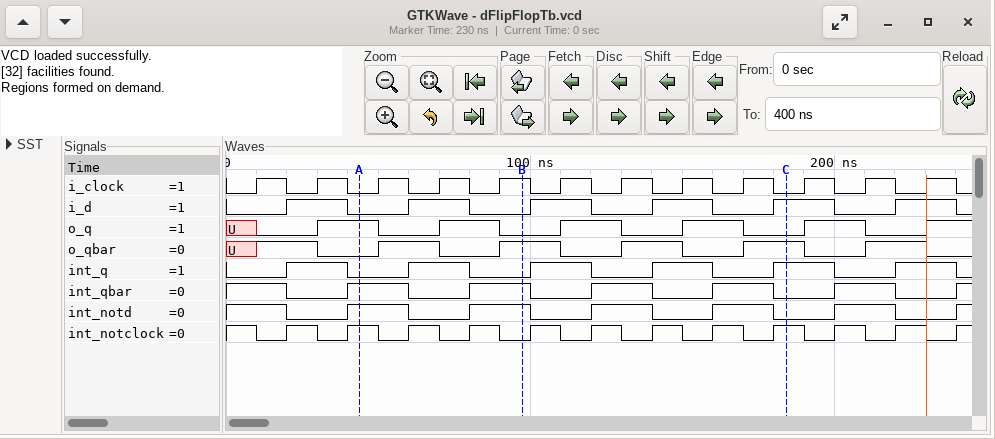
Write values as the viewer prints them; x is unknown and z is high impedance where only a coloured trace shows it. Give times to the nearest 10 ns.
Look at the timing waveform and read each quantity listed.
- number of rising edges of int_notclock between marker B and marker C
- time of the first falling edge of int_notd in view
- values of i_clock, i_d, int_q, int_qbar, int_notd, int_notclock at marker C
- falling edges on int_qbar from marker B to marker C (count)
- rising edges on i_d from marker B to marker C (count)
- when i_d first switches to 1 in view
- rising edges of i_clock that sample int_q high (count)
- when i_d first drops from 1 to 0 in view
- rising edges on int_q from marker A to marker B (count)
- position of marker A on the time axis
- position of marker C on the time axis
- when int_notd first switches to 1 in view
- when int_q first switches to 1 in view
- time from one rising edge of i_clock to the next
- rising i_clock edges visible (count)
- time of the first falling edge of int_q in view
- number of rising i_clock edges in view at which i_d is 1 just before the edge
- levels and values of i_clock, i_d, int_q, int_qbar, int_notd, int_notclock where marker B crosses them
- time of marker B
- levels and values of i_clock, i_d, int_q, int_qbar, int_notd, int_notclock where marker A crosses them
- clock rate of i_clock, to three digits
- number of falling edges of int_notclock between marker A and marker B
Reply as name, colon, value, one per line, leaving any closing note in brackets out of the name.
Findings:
number of rising edges of int_notclock between marker B and marker C: 5
time of the first falling edge of int_notd in view: 20 ns
values of i_clock, i_d, int_q, int_qbar, int_notd, int_notclock at marker C: i_clock=0, i_d=1, int_q=1, int_qbar=0, int_notd=0, int_notclock=1
falling edges on int_qbar from marker B to marker C: 3
rising edges on i_d from marker B to marker C: 3
when i_d first switches to 1 in view: 20 ns
rising edges of i_clock that sample int_q high: 6
when i_d first drops from 1 to 0 in view: 40 ns
rising edges on int_q from marker A to marker B: 1
position of marker A on the time axis: 40 ns
position of marker C on the time axis: 180 ns
when int_notd first switches to 1 in view: 40 ns
when int_q first switches to 1 in view: 20 ns
time from one rising edge of i_clock to the next: 20 ns
rising i_clock edges visible: 12
time of the first falling edge of int_q in view: 40 ns
number of rising i_clock edges in view at which i_d is 1 just before the edge: 6
levels and values of i_clock, i_d, int_q, int_qbar, int_notd, int_notclock where marker B crosses them: i_clock=1, i_d=0, int_q=0, int_qbar=1, int_notd=1, int_notclock=0
time of marker B: 100 ns
levels and values of i_clock, i_d, int_q, int_qbar, int_notd, int_notclock where marker A crosses them: i_clock=0, i_d=0, int_q=0, int_qbar=1, int_notd=1, int_notclock=1
clock rate of i_clock, to three digits: 50.0 MHz
number of falling edges of int_notclock between marker A and marker B: 3
